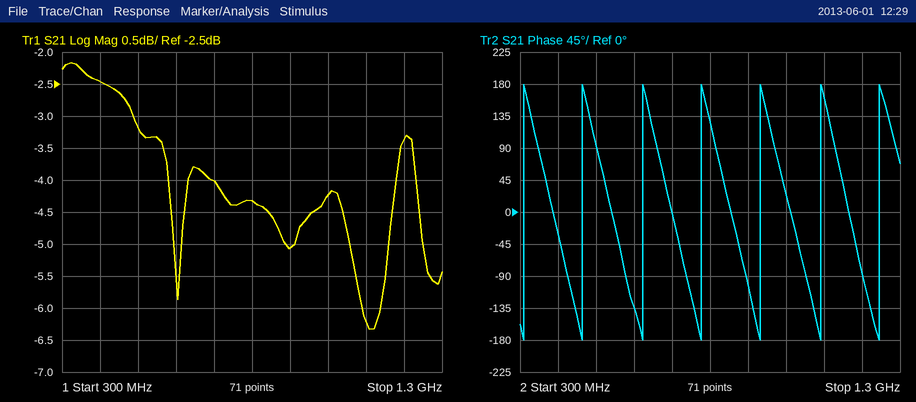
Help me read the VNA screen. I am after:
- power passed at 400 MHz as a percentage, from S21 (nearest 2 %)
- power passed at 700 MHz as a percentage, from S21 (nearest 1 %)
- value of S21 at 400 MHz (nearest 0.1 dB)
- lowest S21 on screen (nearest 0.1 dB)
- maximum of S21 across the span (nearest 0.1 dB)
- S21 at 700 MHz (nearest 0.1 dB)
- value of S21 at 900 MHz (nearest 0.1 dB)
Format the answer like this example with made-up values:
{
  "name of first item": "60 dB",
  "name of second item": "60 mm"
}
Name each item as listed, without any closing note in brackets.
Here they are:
{
  "power passed at 400 MHz as a percentage, from S21": "56 %",
  "power passed at 700 MHz as a percentage, from S21": "40 %",
  "value of S21 at 400 MHz": "-2.5 dB",
  "lowest S21 on screen": "-6.3 dB",
  "maximum of S21 across the span": "-2.2 dB",
  "S21 at 700 MHz": "-4.0 dB",
  "value of S21 at 900 MHz": "-5.1 dB"
}
